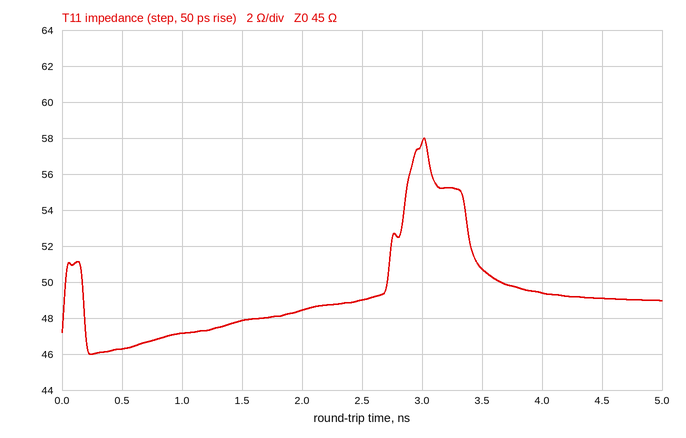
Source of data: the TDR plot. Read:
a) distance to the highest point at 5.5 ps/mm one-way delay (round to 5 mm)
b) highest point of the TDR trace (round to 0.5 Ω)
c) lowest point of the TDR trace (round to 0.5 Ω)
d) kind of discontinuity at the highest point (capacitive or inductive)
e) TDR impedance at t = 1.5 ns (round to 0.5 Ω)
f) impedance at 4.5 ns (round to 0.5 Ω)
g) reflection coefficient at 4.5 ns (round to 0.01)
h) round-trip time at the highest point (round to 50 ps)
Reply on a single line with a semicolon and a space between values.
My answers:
275 mm; 58.0 Ω; 46.0 Ω; inductive; 48.0 Ω; 49.0 Ω; +0.04; 3.00 ns
